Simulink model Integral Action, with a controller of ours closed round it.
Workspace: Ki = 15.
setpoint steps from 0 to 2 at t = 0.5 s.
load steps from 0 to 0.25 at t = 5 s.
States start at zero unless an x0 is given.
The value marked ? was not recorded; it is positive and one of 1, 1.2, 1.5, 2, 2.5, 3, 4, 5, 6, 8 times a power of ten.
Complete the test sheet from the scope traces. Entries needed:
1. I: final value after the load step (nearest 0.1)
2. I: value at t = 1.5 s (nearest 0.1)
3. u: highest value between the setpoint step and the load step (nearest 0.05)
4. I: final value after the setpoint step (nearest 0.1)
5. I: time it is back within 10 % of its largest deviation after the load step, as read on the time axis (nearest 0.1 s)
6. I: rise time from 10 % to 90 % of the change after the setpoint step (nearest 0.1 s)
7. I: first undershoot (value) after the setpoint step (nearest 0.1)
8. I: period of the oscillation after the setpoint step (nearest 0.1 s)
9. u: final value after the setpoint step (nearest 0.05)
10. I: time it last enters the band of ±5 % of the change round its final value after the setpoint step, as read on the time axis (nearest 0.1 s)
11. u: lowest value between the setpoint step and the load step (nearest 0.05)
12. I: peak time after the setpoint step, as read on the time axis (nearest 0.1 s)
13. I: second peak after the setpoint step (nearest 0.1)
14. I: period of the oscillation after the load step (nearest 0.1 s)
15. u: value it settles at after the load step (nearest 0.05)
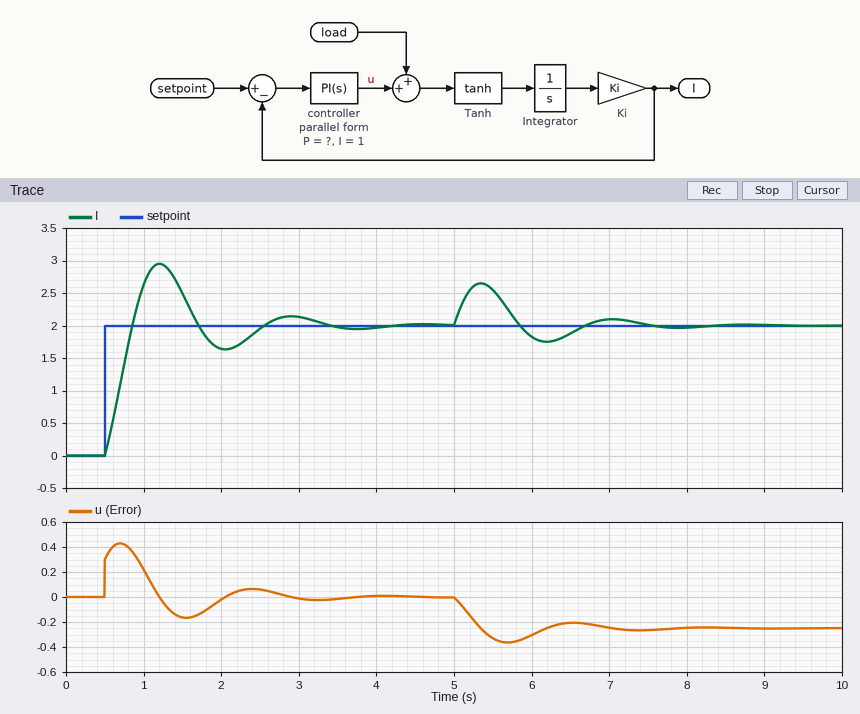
2.0
2.5
0.45
2.0
7.3 s
0.3 s
1.6
1.7 s
0.00
3.1 s
-0.15
1.2 s
2.1
1.7 s
-0.25
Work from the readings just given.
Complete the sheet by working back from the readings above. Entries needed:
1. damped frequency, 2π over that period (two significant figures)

3.7 rad/s
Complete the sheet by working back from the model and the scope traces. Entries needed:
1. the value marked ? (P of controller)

0.15
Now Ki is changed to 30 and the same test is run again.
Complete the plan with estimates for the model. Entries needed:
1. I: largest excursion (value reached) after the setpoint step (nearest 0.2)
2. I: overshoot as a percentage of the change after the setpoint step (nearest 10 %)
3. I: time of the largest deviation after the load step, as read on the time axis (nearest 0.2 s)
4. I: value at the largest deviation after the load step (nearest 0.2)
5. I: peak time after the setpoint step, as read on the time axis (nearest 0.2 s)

2.8
40 %
5.2 s
2.8
1.0 s
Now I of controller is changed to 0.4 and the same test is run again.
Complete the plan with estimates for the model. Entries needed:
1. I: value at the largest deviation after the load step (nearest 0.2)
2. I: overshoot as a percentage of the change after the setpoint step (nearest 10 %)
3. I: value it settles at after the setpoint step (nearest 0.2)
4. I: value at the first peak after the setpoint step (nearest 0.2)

2.8
30 %
2.0
2.6
